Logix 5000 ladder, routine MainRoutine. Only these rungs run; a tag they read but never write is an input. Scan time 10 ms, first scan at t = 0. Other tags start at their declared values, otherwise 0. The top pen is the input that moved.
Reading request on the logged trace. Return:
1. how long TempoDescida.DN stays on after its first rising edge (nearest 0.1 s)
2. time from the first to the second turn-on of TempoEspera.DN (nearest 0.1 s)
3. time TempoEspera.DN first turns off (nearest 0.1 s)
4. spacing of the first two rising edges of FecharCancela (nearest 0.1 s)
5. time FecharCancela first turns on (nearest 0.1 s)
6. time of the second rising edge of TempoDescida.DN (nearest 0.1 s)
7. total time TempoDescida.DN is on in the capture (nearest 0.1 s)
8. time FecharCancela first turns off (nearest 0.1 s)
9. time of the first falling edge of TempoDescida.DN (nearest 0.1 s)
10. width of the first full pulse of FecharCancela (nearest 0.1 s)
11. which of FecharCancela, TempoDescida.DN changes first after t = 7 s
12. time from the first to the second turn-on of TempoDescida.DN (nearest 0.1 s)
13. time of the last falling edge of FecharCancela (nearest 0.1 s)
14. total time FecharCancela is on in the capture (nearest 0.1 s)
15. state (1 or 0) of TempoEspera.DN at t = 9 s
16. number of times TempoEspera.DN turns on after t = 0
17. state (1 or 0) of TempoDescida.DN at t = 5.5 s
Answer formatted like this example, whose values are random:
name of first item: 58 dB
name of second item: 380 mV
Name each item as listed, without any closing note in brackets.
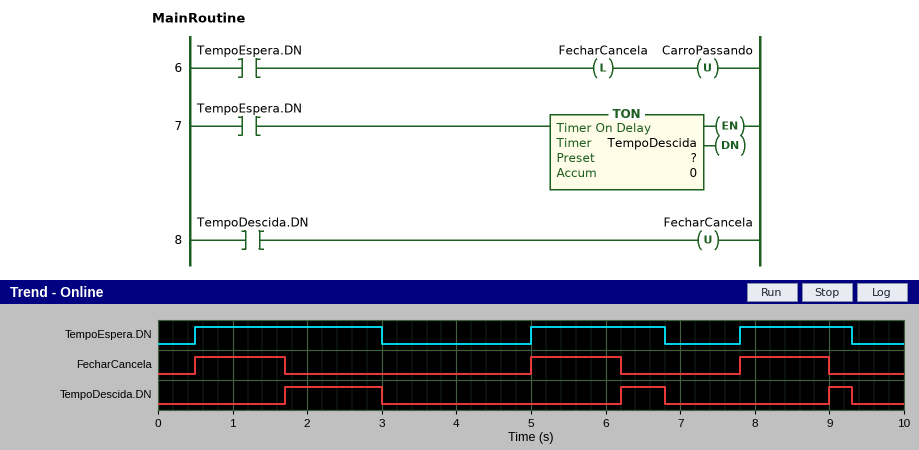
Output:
how long TempoDescida.DN stays on after its first rising edge: 1.3 s
time from the first to the second turn-on of TempoEspera.DN: 4.5 s
time TempoEspera.DN first turns off: 3.0 s
spacing of the first two rising edges of FecharCancela: 4.5 s
time FecharCancela first turns on: 0.5 s
time of the second rising edge of TempoDescida.DN: 6.2 s
total time TempoDescida.DN is on in the capture: 2.2 s
time FecharCancela first turns off: 1.7 s
time of the first falling edge of TempoDescida.DN: 3.0 s
width of the first full pulse of FecharCancela: 1.2 s
which of FecharCancela, TempoDescida.DN changes first after t = 7 s: FecharCancela
time from the first to the second turn-on of TempoDescida.DN: 4.5 s
time of the last falling edge of FecharCancela: 9.0 s
total time FecharCancela is on in the capture: 3.6 s
state (1 or 0) of TempoEspera.DN at t = 9 s: 1
number of times TempoEspera.DN turns on after t = 0: 3
state (1 or 0) of TempoDescida.DN at t = 5.5 s: 0
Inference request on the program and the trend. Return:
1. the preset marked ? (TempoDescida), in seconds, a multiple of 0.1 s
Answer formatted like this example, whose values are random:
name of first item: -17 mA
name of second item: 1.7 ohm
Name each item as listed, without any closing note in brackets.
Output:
the preset marked ? (TempoDescida), in seconds, a multiple of 0.1 s: 1.2 s
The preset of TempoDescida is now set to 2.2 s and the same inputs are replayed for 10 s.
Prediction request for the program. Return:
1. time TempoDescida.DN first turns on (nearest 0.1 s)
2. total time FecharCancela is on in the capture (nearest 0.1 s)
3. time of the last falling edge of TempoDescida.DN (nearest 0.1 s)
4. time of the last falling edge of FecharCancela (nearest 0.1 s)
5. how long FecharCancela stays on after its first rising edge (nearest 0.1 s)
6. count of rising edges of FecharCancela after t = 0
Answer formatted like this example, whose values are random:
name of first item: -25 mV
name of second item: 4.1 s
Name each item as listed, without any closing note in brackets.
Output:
time TempoDescida.DN first turns on: 2.7 s
total time FecharCancela is on in the capture: 7.2 s
time of the last falling edge of TempoDescida.DN: 3.0 s
time of the last falling edge of FecharCancela: 2.7 s
how long FecharCancela stays on after its first rising edge: 2.2 s
count of rising edges of FecharCancela after t = 0: 2
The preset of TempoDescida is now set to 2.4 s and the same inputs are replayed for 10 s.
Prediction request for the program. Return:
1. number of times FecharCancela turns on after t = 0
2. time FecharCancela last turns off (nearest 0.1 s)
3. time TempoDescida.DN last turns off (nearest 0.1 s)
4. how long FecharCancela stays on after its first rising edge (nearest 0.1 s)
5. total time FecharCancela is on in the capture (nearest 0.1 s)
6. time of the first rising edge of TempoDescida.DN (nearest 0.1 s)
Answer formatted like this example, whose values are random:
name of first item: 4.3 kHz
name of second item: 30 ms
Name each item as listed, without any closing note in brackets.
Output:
number of times FecharCancela turns on after t = 0: 2
time FecharCancela last turns off: 2.9 s
time TempoDescida.DN last turns off: 3.0 s
how long FecharCancela stays on after its first rising edge: 2.4 s
total time FecharCancela is on in the capture: 7.4 s
time of the first rising edge of TempoDescida.DN: 2.9 s
